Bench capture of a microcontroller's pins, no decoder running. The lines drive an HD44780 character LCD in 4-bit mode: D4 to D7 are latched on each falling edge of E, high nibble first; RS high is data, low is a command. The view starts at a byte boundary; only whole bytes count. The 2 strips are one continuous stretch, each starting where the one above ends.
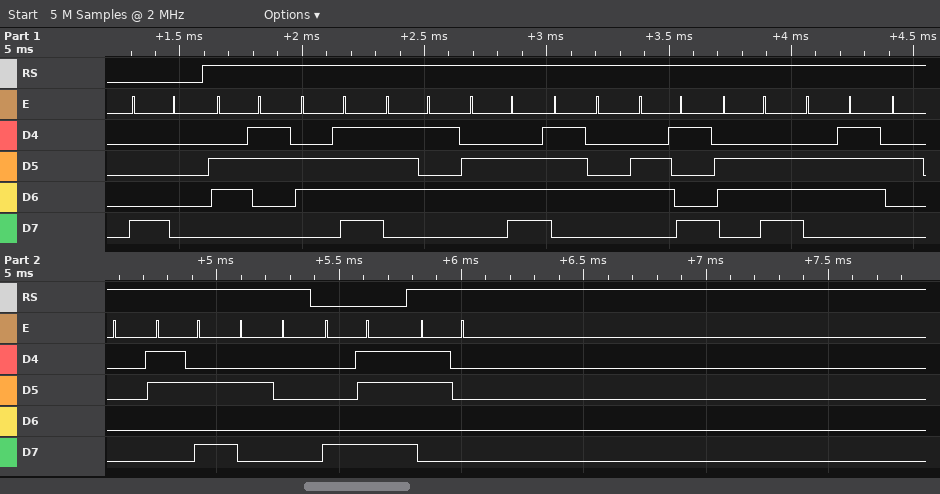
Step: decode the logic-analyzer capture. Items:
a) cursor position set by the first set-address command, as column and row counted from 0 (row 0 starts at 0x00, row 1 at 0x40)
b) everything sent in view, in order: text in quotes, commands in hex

column 0, row 0
0x80 "counting : " 0x8B "0"
